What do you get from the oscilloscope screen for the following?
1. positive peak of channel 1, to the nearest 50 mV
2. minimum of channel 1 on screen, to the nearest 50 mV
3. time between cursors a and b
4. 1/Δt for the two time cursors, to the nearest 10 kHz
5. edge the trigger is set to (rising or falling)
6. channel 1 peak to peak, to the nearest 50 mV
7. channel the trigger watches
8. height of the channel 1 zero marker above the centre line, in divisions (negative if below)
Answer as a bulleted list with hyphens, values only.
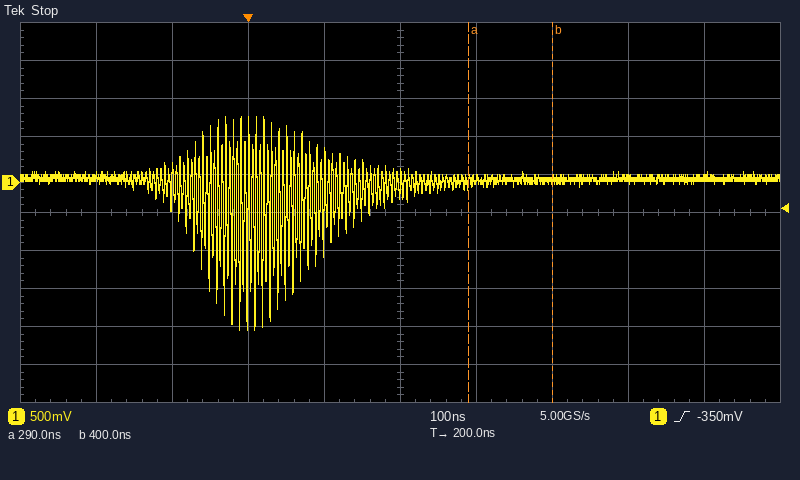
- 850 mV
- -1.95 V
- 110 ns
- 9.09 MHz
- rising
- 2.80 V
- channel 1
- +0.8 div
